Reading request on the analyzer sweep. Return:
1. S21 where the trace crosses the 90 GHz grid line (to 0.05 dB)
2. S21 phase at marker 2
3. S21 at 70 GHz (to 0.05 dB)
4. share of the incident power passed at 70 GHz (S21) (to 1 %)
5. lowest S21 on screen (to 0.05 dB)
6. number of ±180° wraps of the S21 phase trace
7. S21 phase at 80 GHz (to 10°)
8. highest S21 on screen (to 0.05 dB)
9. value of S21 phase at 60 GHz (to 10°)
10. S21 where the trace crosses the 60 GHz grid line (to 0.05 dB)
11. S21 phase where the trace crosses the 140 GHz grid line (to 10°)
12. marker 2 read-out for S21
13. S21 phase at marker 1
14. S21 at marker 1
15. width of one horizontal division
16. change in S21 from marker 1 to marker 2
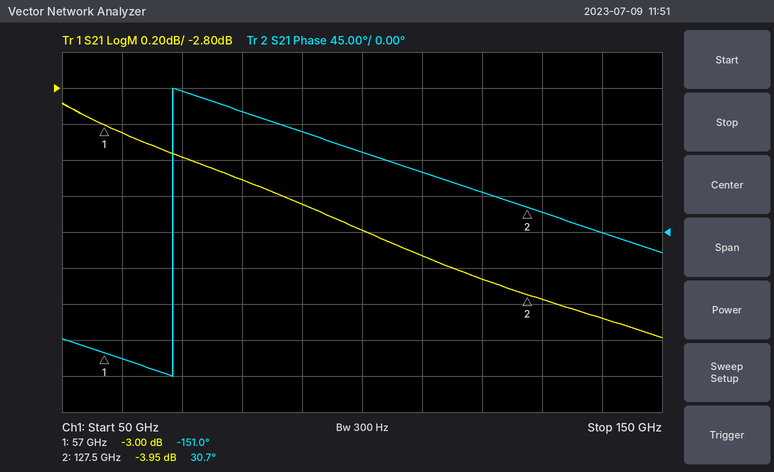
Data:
-3.45 dB
30.7°
-3.20 dB
48 %
-4.20 dB
1
150°
-2.90 dB
-160°
-3.05 dB
0°
-3.95 dB
-151.0°
-3.00 dB
10 GHz
-0.95 dB
